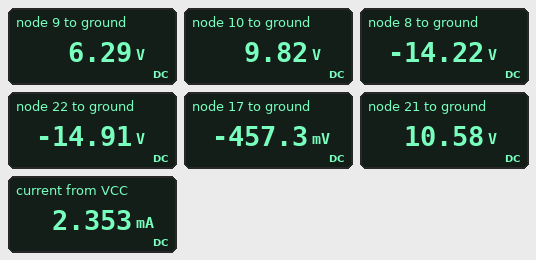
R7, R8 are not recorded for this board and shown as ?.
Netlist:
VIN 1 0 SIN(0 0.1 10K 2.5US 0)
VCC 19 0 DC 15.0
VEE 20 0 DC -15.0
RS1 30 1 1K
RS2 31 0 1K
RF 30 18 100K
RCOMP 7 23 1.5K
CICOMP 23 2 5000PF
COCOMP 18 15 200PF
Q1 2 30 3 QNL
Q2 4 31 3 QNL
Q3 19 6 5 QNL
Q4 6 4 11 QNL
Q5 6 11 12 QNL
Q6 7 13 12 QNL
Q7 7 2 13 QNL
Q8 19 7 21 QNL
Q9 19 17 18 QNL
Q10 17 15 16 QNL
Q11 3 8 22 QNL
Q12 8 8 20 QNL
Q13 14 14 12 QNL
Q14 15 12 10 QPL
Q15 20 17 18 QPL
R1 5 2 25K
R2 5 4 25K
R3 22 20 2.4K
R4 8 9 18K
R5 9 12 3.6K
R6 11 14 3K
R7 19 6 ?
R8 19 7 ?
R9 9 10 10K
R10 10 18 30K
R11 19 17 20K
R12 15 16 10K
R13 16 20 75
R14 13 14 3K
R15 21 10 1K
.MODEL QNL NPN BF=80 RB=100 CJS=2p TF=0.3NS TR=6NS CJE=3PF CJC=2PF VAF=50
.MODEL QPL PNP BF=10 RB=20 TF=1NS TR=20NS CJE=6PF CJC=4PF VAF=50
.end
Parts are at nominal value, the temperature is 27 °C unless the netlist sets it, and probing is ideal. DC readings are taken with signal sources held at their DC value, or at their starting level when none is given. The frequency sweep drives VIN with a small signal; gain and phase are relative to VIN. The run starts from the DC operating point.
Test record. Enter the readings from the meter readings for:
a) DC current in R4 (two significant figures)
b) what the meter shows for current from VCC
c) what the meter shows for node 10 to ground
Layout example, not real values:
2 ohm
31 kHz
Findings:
1.1 mA
2.353 mA
9.82 V
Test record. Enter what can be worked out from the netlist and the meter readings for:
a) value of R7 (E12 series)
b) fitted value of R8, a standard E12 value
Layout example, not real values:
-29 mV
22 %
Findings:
5.6 kΩ
18 kΩ
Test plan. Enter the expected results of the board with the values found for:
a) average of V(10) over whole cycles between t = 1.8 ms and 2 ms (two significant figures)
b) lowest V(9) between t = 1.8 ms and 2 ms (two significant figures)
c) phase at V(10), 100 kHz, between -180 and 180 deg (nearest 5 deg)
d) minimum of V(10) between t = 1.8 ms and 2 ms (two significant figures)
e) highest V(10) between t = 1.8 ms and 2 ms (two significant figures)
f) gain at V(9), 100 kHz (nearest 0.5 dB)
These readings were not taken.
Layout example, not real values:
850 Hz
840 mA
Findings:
9.8 V
6.1 V
0 deg
9.6 V
10 V
10.0 dB
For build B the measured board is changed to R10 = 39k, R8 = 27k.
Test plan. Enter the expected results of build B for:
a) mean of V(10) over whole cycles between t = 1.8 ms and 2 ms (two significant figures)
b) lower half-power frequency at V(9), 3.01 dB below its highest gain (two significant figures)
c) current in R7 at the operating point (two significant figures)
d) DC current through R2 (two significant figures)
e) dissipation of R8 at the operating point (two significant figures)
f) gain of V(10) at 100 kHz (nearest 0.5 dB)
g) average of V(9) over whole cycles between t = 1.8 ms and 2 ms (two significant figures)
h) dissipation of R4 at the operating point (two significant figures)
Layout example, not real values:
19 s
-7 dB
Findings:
9.6 V
6.5 kHz
630 µA
18 µA
590 µW
12.0 dB
6.1 V
23 mW
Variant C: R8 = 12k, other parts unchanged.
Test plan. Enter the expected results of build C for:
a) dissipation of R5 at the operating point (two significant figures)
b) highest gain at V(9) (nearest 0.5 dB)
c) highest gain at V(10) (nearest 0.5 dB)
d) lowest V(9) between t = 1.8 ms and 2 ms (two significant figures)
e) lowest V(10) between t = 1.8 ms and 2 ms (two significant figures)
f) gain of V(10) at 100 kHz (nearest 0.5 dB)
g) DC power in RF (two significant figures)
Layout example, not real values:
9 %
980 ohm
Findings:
2.3 mW
9.5 dB
11.0 dB
6.4 V
10 V
10.5 dB
280 nW
